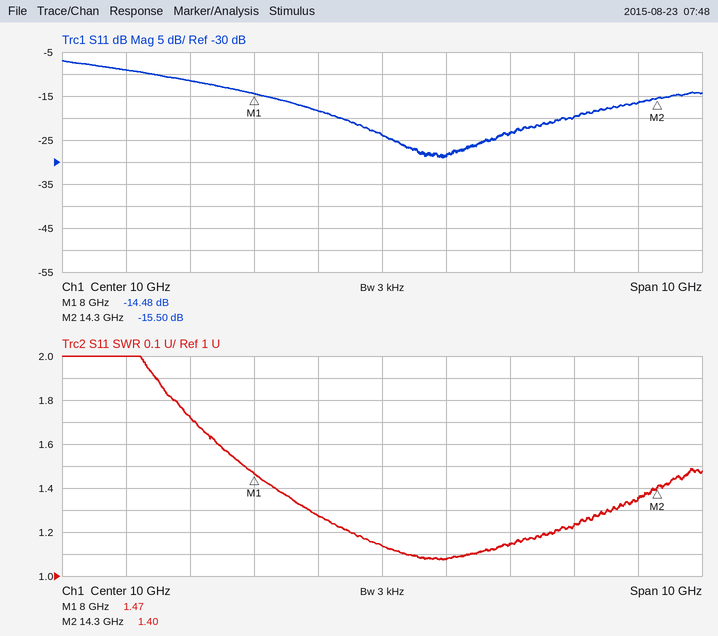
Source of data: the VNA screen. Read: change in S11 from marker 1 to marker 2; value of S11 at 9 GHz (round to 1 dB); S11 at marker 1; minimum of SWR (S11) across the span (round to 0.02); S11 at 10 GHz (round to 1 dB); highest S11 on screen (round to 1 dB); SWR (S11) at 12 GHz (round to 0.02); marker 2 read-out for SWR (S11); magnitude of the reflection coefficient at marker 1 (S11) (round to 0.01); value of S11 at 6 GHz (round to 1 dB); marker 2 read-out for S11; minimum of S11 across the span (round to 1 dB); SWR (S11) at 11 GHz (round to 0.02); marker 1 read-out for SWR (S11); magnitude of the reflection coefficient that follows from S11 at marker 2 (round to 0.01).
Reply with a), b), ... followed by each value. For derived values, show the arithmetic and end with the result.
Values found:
a) -15.5 − (-14.48) = -1.02 dB
b) -18 dB
c) -14.48 dB
d) 1.08
e) -24 dB
f) -7 dB
g) 1.14
h) 1.40
i) 10^(-14.48/20) ≈ 0.19
j) -9 dB
k) -15.50 dB
l) -29 dB
m) 1.08
n) 1.47
o) 10^(-15.5/20) ≈ 0.17
